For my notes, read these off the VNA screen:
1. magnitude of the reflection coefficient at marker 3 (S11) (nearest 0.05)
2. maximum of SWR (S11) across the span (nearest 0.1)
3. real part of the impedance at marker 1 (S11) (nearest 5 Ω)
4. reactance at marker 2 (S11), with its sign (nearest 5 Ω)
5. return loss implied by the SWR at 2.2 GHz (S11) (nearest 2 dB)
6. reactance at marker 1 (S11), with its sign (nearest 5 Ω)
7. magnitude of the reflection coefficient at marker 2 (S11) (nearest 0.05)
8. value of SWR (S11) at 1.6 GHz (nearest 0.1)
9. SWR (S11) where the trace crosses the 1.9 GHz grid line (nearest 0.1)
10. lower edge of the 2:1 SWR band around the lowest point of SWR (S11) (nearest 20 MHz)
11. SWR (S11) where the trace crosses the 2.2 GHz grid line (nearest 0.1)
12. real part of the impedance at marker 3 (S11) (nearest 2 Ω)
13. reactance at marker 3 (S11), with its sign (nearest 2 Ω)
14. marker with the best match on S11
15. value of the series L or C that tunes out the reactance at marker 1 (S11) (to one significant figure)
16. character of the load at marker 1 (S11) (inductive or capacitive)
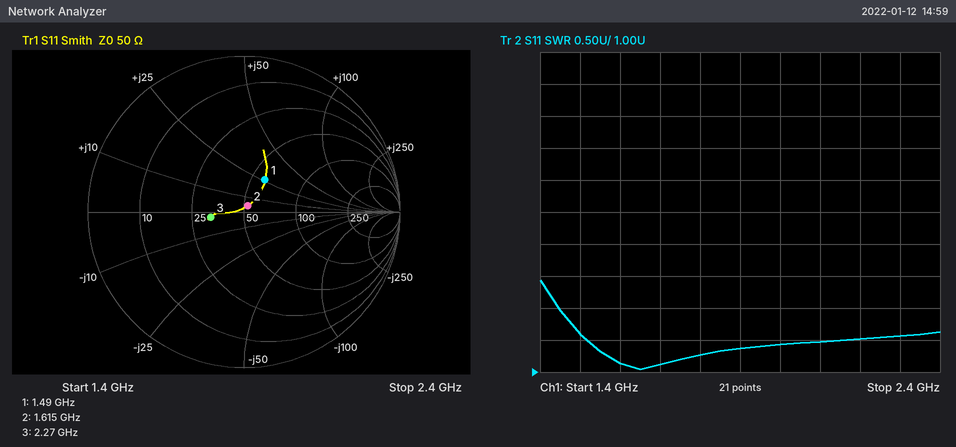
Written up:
0.20
2.4
60 Ω
+5 Ω
14 dB
+25 Ω
0.05
1.1
1.4
1.44 GHz
1.5
32 Ω
-2 Ω
marker 2
4 pF
inductive
